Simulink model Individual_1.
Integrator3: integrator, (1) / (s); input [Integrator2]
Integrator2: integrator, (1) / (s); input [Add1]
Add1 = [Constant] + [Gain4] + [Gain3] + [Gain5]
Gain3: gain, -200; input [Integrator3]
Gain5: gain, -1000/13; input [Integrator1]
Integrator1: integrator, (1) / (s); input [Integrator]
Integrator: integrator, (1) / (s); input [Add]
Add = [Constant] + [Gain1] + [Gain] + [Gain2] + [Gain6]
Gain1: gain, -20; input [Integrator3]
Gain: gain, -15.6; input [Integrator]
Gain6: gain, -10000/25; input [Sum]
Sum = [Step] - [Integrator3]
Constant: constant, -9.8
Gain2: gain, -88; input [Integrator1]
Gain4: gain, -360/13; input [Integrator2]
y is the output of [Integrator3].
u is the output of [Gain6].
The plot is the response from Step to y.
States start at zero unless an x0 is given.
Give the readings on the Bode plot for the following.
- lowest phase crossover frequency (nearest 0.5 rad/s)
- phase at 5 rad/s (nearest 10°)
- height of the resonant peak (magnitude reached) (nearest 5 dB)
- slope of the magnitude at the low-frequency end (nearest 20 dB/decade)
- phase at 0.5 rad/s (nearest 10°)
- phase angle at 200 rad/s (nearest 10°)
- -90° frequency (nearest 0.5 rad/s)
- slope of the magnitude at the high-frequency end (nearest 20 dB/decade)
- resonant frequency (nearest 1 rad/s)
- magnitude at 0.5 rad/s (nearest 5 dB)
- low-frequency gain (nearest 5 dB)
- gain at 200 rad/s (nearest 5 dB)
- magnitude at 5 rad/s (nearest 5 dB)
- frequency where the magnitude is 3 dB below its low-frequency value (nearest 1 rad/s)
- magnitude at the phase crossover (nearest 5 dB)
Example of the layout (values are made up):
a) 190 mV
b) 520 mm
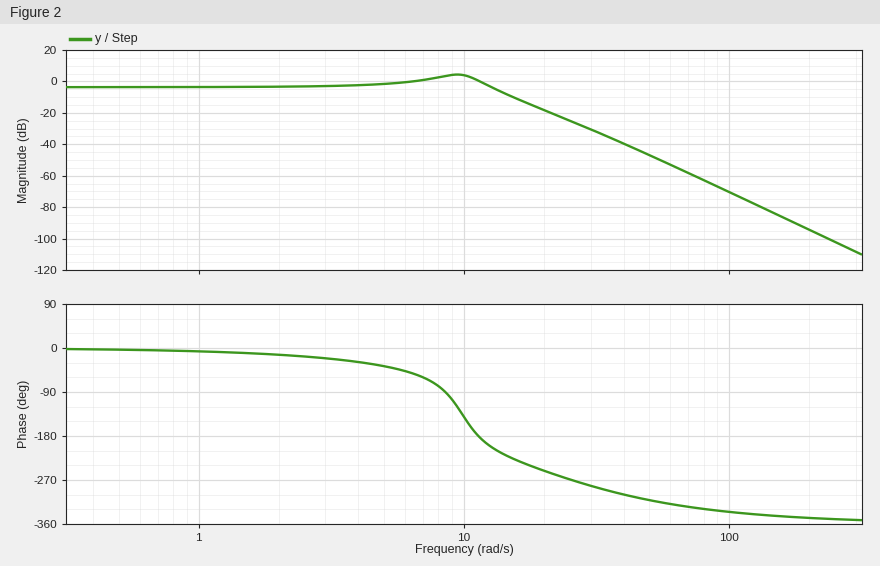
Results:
a) 11.5 rad/s
b) -40°
c) 5 dB
d) 0 dB/decade
e) 0°
f) -350°
g) 8.5 rad/s
h) -80 dB/decade
i) 9 rad/s
j) -5 dB
k) -5 dB
l) -95 dB
m) 0 dB
n) 14 rad/s
o) 0 dB
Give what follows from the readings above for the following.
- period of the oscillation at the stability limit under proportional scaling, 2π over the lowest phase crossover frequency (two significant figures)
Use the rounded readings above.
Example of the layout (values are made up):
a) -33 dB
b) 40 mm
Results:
a) 0.55 s
